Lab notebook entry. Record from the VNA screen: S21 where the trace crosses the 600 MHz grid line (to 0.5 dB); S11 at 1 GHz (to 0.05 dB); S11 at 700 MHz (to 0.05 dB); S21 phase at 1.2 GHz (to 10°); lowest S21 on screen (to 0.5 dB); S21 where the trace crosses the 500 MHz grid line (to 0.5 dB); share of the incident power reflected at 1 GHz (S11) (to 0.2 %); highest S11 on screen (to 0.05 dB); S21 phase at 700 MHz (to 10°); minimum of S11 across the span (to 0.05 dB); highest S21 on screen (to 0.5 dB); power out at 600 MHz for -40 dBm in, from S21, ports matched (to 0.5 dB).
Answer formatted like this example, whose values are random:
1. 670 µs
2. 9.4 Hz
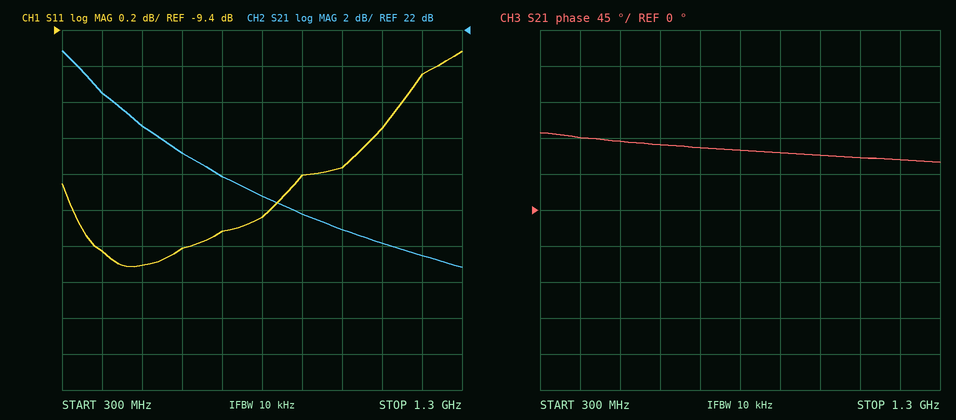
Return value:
1. 15.0 dB
2. -10.15 dB
3. -10.50 dB
4. 60°
5. 9.0 dB
6. 16.5 dB
7. 9.6 %
8. -9.50 dB
9. 80°
10. -10.70 dB
11. 21.0 dB
12. -25.0 dBm
